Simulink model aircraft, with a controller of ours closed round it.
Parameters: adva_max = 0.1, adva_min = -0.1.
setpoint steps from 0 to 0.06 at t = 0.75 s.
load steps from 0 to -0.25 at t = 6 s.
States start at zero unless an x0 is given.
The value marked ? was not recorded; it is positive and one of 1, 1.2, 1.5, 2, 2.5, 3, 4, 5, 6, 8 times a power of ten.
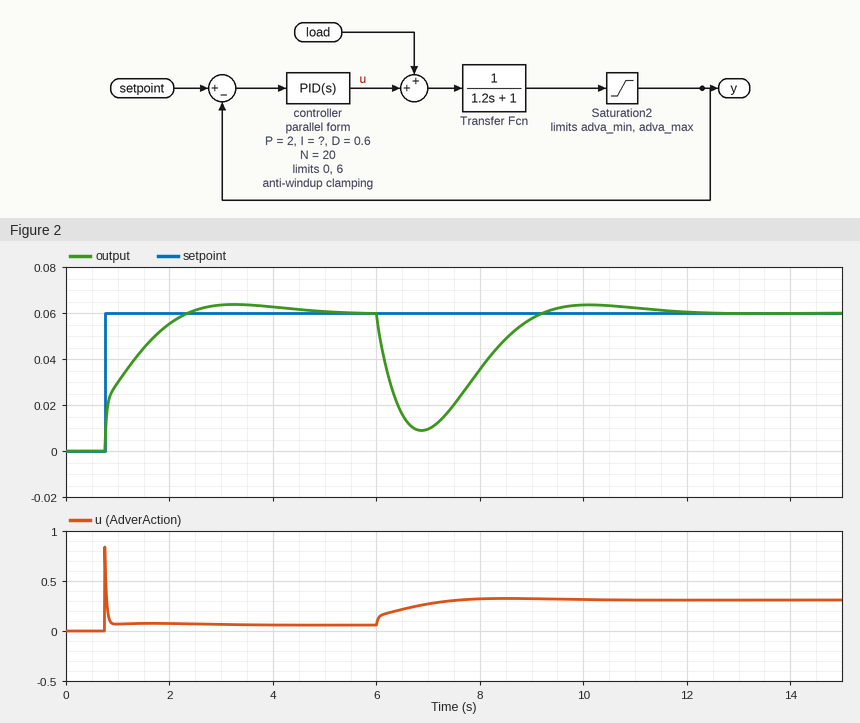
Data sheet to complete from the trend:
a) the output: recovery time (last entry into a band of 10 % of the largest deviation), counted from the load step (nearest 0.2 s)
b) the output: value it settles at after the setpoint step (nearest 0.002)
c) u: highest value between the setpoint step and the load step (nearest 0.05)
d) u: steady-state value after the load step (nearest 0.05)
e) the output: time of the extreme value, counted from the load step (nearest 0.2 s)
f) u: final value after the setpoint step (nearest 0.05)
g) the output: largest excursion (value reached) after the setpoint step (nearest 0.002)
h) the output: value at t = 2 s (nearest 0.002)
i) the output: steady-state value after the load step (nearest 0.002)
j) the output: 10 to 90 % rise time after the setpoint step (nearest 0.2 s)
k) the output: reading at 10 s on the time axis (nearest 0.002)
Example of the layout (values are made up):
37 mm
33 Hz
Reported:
2.8 s
0.060
0.85
0.30
0.8 s
0.05
0.064
0.056
0.060
1.2 s
0.064
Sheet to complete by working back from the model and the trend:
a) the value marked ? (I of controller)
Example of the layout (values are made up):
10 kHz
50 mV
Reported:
3
